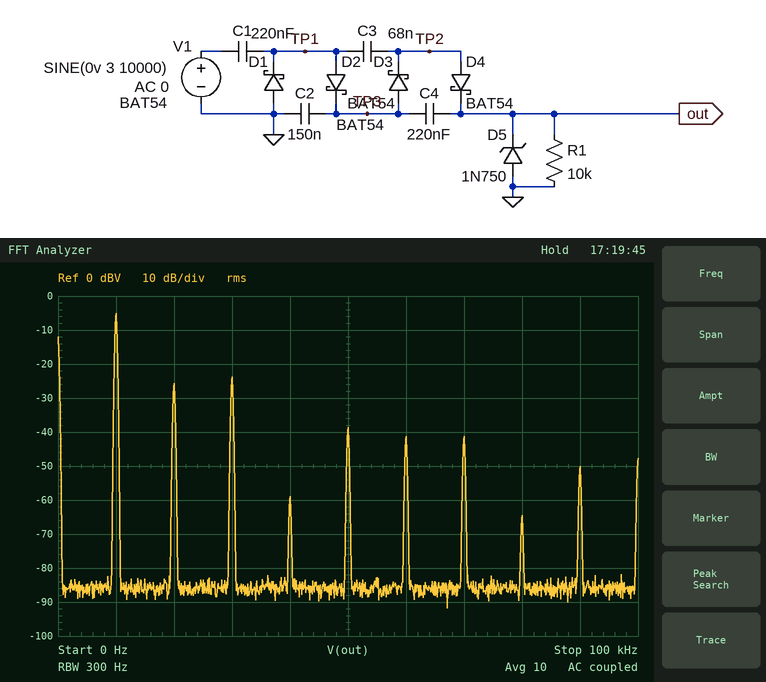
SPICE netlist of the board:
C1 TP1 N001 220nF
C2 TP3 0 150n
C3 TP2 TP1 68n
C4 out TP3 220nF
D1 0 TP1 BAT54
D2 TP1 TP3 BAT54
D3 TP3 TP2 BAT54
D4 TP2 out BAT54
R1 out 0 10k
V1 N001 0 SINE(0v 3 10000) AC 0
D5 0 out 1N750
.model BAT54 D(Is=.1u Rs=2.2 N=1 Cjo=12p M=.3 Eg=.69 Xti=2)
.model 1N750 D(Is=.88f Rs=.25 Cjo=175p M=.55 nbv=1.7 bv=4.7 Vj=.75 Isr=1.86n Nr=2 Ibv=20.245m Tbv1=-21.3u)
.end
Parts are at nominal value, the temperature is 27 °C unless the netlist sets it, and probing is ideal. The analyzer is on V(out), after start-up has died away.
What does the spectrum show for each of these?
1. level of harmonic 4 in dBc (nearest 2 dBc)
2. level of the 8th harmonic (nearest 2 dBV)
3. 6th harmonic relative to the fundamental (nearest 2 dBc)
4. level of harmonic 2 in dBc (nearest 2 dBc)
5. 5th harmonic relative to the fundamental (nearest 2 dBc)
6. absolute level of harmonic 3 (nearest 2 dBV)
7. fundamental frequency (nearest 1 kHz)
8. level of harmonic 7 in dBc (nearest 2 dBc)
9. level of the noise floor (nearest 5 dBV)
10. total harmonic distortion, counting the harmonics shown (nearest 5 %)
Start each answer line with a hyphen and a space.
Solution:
- -54 dBc
- -64 dBV
- -36 dBc
- -20 dBc
- -34 dBc
- -24 dBV
- 10 kHz
- -36 dBc
- -85 dBV
- 15 %
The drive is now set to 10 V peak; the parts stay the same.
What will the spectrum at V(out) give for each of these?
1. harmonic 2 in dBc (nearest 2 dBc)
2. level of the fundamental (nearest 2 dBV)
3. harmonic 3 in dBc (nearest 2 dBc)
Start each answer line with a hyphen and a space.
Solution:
- -24 dBc
- -2 dBV
- -14 dBc
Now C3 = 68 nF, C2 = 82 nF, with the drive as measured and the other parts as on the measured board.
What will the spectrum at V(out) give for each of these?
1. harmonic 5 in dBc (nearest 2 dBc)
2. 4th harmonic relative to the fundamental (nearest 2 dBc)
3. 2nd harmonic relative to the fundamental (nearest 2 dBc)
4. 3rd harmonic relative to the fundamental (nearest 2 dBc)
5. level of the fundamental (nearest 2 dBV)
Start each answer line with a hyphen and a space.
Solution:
- -30 dBc
- -36 dBc
- -26 dBc
- -22 dBc
- -2 dBV
